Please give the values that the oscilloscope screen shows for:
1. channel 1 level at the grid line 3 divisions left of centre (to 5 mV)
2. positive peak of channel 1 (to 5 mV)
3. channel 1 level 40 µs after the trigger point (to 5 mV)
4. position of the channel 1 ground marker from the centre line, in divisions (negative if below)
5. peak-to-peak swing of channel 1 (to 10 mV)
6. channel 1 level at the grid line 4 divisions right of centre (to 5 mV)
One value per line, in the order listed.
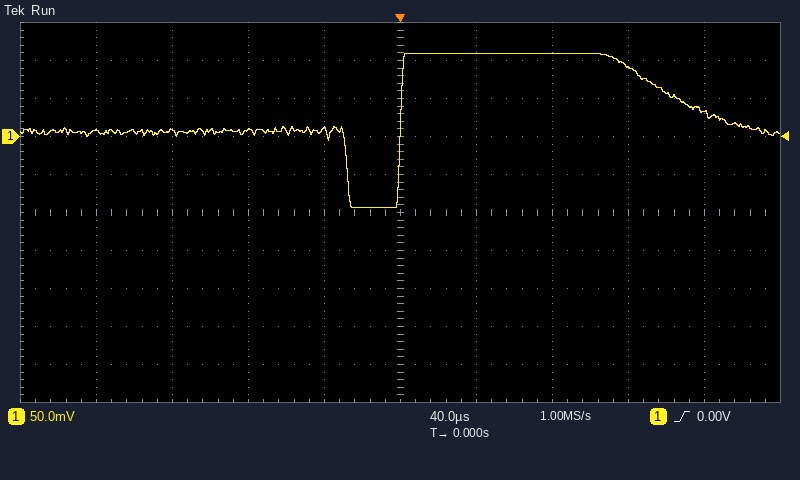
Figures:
5 mV
110 mV
110 mV
+2.0 div
200 mV
30 mV
